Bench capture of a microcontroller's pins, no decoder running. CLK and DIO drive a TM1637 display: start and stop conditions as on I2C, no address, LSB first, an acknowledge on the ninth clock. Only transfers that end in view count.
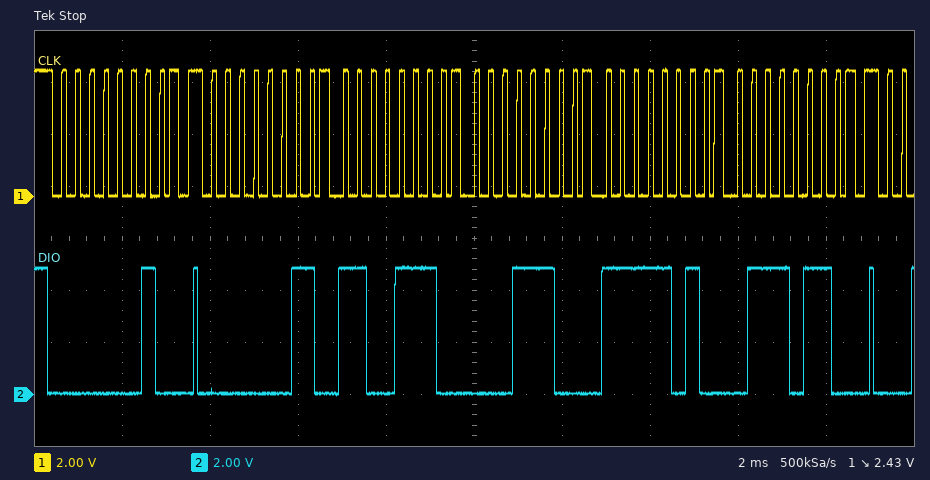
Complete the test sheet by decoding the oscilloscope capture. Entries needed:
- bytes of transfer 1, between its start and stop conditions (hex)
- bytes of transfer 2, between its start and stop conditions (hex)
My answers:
40
C0 73 38 5F 6E
